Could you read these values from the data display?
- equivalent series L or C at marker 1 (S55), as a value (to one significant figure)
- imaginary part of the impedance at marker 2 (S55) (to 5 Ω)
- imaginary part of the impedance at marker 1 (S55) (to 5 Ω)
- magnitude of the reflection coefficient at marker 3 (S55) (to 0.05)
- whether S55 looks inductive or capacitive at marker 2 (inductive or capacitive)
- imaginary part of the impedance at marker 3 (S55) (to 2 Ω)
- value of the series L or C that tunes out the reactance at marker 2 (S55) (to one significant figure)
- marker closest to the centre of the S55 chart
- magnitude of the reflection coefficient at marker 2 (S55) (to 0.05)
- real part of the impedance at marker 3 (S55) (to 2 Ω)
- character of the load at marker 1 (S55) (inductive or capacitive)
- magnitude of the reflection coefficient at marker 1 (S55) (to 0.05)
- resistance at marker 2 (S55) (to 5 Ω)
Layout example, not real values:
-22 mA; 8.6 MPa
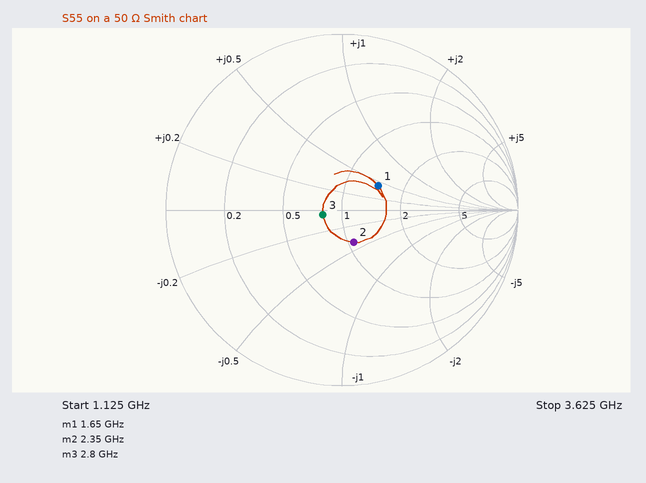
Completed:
2 nH; -20 Ω; +20 Ω; 0.10; capacitive; -2 Ω; 1 nH; marker 3; 0.20; 40 Ω; inductive; 0.25; 55 Ω
